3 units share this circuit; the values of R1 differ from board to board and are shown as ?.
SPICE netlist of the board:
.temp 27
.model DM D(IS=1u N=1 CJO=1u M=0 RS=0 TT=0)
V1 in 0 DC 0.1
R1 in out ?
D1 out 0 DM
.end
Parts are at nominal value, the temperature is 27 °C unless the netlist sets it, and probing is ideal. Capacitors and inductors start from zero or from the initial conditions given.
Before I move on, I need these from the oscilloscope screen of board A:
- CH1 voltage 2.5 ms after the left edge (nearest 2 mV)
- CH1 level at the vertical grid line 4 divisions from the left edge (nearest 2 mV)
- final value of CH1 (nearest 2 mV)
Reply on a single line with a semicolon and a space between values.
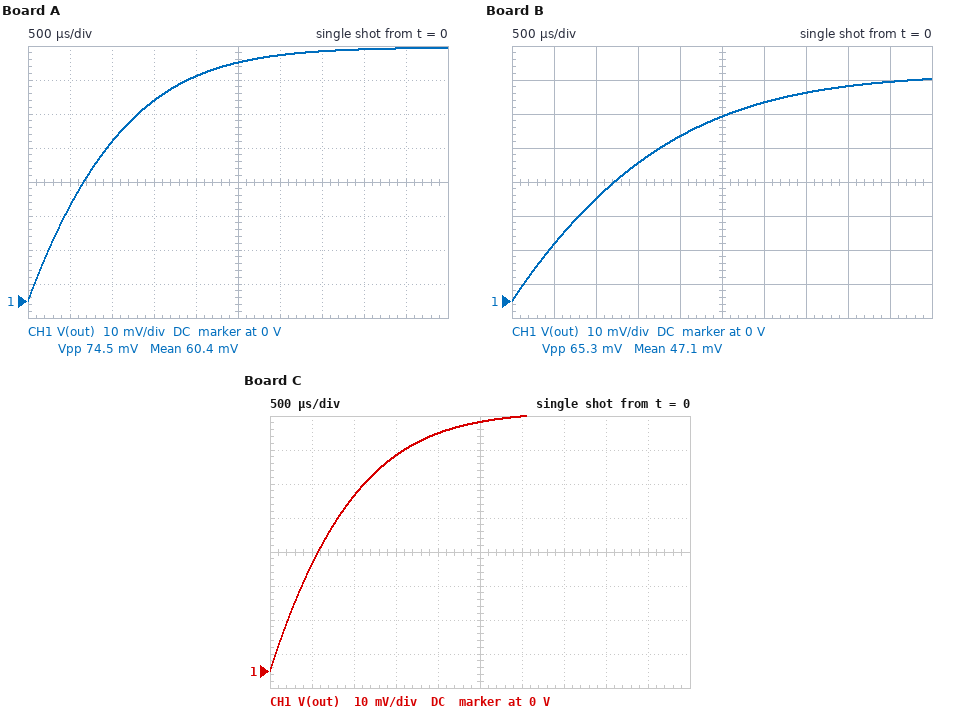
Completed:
70 mV; 66 mV; 74 mV
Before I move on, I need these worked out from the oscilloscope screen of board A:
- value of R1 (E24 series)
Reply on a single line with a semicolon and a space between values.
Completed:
1.5 kΩ
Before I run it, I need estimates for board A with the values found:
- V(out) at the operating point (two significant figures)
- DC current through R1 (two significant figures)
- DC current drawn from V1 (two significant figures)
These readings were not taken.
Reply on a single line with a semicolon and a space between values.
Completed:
75 mV; 17 µA; 17 µA
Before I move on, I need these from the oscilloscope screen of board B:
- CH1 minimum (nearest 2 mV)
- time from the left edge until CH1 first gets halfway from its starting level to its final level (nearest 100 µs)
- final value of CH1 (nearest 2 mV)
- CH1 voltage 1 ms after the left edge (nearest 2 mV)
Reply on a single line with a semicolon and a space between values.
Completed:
0 V; 1.1 ms; 66 mV; 30 mV
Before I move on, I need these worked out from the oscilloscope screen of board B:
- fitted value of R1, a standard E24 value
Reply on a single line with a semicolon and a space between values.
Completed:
2.7 kΩ
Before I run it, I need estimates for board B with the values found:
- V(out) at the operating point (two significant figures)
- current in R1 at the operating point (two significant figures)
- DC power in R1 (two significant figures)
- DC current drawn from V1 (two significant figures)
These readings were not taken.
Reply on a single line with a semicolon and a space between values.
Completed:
67 mV; 12 µA; 410 nW; 12 µA
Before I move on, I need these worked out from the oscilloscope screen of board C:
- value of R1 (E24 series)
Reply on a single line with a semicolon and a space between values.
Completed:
1.3 kΩ
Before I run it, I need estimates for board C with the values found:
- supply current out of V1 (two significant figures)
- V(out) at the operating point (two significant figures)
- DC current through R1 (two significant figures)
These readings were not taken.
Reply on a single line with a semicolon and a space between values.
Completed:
18 µA; 76 mV; 18 µA
